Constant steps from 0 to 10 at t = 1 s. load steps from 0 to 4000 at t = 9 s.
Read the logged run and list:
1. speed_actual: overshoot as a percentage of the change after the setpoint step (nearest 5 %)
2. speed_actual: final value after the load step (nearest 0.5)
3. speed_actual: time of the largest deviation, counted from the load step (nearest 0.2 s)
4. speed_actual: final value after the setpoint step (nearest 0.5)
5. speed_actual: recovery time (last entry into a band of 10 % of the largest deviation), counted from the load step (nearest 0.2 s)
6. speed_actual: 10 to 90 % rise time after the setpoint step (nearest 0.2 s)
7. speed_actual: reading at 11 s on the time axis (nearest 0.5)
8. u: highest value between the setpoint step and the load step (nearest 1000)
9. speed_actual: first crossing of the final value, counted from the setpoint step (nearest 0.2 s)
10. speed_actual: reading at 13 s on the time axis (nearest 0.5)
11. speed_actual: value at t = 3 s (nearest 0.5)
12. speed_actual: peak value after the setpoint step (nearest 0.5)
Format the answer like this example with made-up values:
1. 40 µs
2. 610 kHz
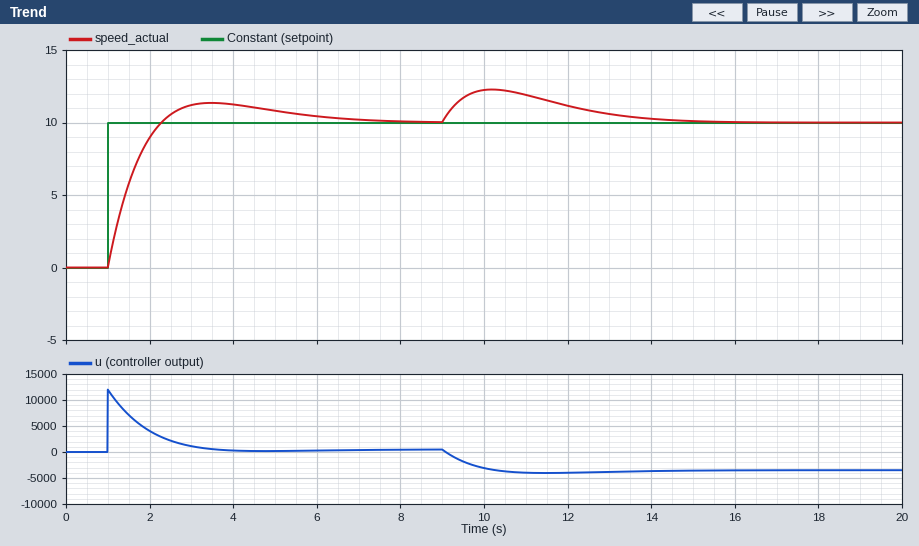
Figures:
1. 15 %
2. 10.0
3. 1.2 s
4. 10.0
5. 5.2 s
6. 1.0 s
7. 12.0
8. 12000
9. 1.2 s
10. 10.5
11. 11.0
12. 11.5
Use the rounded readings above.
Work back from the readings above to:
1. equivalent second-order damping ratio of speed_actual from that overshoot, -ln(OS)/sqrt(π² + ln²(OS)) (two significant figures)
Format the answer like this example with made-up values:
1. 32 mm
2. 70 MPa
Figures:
1. 0.52
